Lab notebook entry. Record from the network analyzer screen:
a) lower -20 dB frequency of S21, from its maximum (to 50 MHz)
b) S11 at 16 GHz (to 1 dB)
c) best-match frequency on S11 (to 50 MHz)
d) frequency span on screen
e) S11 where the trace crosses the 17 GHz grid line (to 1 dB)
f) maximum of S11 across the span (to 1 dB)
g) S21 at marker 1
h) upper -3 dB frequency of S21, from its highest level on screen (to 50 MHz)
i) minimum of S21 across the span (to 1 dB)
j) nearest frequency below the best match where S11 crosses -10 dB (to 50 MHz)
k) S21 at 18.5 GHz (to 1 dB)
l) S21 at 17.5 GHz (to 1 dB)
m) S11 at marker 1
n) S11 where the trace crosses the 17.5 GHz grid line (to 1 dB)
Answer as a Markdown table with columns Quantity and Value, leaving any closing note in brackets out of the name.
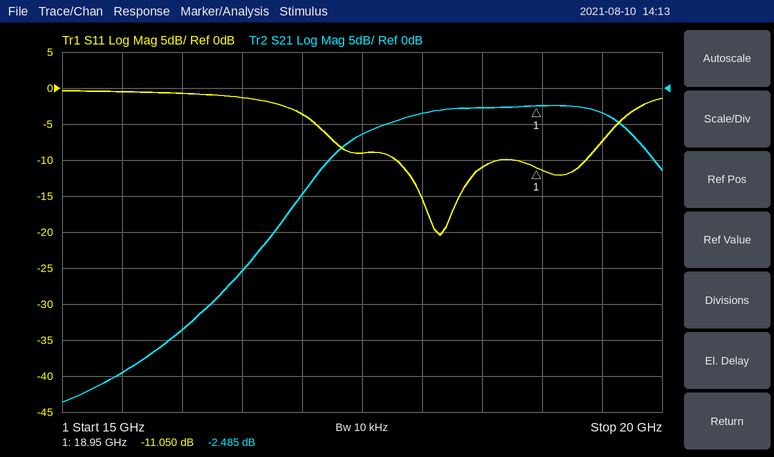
| Quantity | Value |
|---|---|
| lower -20 dB frequency of S21, from its maximum | 16.65 GHz |
| S11 at 16 GHz | -1 dB |
| best-match frequency on S11 | 18.15 GHz |
| frequency span on screen | 5 GHz |
| S11 where the trace crosses the 17 GHz grid line | -4 dB |
| maximum of S11 across the span | 0 dB |
| S21 at marker 1 | -2.485 dB |
| upper -3 dB frequency of S21, from its highest level on screen | 19.70 GHz |
| minimum of S21 across the span | -44 dB |
| nearest frequency below the best match where S11 crosses -10 dB | 17.80 GHz |
| S21 at 18.5 GHz | -3 dB |
| S21 at 17.5 GHz | -6 dB |
| S11 at marker 1 | -11.050 dB |
| S11 where the trace crosses the 17.5 GHz grid line | -9 dB |
